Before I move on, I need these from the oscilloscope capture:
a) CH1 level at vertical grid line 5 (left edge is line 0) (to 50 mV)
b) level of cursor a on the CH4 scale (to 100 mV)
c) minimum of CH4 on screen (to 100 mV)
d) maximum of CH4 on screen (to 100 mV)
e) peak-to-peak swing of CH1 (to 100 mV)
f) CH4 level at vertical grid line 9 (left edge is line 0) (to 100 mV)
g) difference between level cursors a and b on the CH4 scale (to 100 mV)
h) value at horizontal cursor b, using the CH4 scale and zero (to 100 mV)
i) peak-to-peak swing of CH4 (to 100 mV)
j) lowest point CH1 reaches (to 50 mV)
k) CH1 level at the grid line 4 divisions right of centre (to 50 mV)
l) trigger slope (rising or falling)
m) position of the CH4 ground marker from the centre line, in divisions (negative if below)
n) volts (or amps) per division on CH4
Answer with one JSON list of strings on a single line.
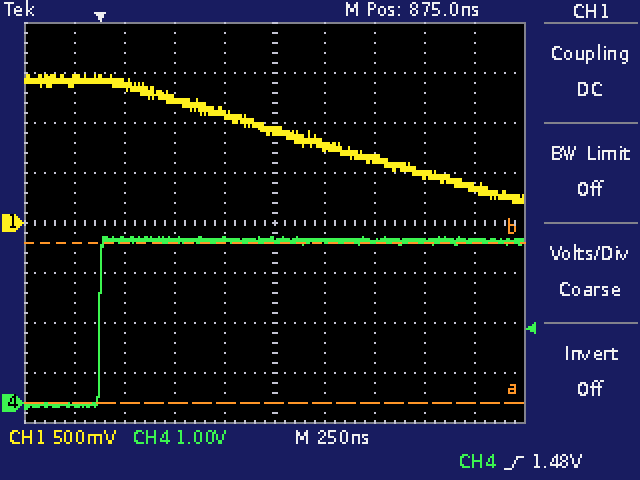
["900 mV", "0.0 V", "-100 mV", "3.3 V", "1.30 V", "3.2 V", "3.2 V", "3.2 V", "3.4 V", "200 mV", "350 mV", "rising", "-3.6 div", "1 V"]
